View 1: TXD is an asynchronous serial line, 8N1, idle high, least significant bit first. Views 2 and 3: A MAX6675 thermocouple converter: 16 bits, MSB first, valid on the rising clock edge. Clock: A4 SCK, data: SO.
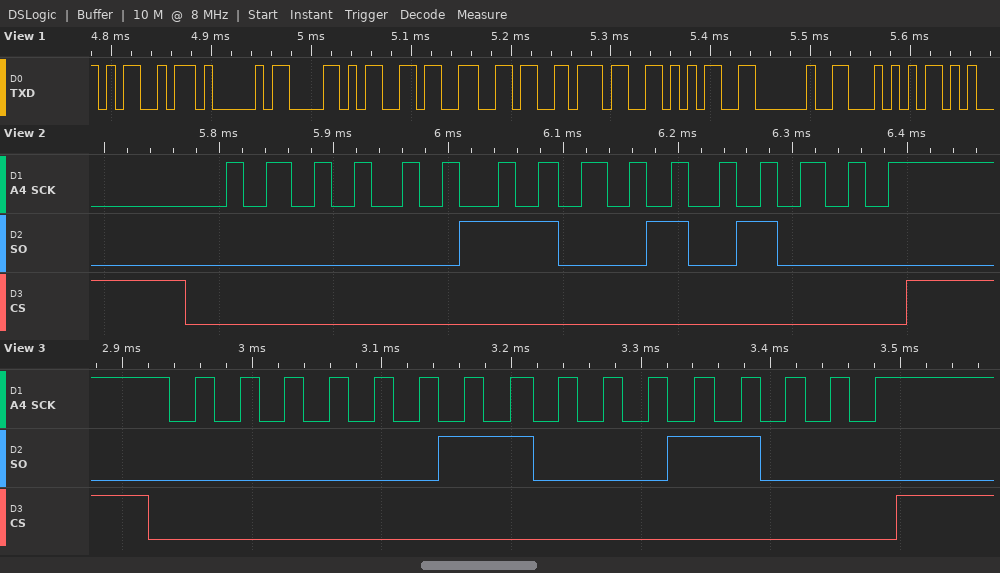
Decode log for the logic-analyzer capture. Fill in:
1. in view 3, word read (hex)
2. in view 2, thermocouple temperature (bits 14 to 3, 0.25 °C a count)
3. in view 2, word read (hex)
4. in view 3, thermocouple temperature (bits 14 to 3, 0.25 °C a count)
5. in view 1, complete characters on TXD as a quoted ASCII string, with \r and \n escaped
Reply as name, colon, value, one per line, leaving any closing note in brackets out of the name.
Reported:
in view 3, word read: 0x0318
in view 2, thermocouple temperature: 25.25 °C
in view 2, word read: 0x0328
in view 3, thermocouple temperature: 24.75 °C
in view 1, complete characters on TXD as a quoted ASCII string, with \r and \n escaped: "MAX6675 T"
